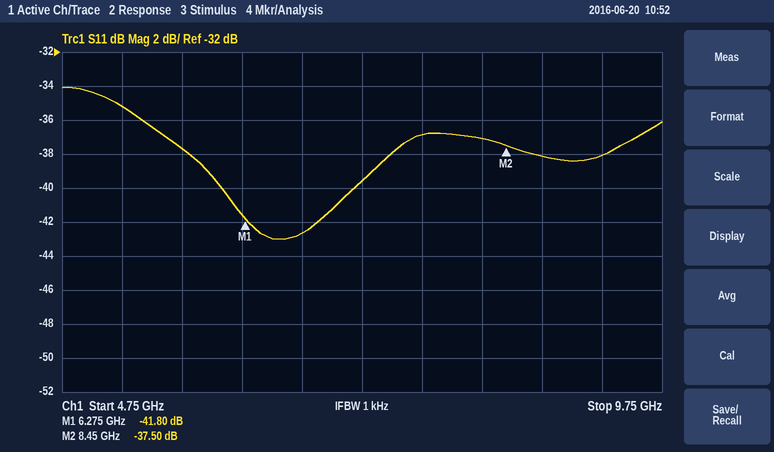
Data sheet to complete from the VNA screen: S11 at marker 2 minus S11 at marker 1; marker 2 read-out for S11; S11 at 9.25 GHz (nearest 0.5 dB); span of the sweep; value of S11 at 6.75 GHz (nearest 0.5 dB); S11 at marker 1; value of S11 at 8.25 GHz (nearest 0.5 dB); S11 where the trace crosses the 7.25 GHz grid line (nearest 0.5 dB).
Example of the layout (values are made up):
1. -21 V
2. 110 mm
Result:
1. 4.30 dB
2. -37.50 dB
3. -38.0 dB
4. 5 GHz
5. -42.5 dB
6. -41.80 dB
7. -37.0 dB
8. -39.5 dB
